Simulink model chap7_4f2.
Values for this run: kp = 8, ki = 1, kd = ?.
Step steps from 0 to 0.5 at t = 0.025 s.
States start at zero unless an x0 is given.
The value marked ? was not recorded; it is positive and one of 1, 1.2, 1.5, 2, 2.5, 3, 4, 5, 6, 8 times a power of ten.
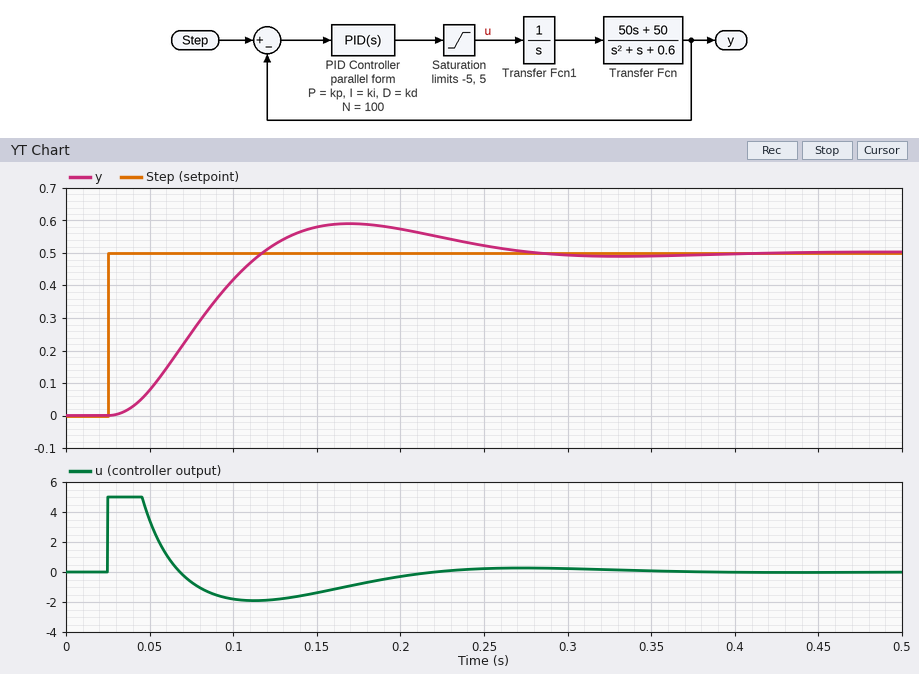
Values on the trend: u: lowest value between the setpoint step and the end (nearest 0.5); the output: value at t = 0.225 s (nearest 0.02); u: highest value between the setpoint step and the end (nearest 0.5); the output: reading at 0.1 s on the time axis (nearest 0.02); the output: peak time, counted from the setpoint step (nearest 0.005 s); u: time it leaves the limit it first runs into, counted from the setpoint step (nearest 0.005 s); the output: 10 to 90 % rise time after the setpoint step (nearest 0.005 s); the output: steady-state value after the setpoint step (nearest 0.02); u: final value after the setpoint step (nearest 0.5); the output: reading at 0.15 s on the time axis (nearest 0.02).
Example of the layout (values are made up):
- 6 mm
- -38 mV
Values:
- -2.0
- 0.54
- 5.0
- 0.42
- 0.145 s
- 0.020 s
- 0.060 s
- 0.50
- 0.0
- 0.58
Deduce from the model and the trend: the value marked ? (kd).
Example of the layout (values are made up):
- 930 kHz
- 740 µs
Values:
- 0.4
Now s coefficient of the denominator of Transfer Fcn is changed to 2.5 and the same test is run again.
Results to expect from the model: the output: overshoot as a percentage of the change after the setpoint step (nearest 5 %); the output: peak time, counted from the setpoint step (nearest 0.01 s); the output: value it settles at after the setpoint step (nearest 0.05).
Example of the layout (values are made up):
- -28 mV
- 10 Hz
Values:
- 15 %
- 0.15 s
- 0.50
